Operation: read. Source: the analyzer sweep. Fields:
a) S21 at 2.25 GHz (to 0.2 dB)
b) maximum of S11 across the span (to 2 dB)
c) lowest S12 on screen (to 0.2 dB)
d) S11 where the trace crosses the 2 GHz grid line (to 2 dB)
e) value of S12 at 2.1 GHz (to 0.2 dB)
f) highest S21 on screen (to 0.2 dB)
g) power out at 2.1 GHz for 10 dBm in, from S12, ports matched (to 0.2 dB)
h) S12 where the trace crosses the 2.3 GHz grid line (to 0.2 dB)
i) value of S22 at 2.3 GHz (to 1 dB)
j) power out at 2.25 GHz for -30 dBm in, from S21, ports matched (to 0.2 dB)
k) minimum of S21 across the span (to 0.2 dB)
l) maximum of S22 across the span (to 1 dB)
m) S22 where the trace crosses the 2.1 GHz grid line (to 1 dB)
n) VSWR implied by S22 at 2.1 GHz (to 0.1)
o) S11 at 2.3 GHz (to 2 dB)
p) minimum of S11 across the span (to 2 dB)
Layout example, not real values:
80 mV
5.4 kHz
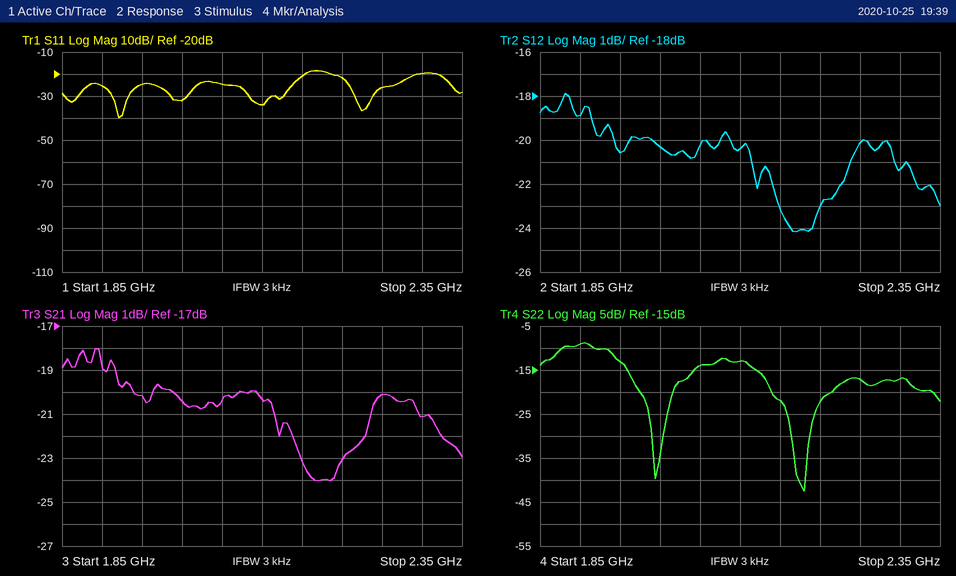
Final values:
-20.2 dB
-18 dB
-24.2 dB
-32 dB
-20.4 dB
-18.0 dB
-10.4 dBm
-21.4 dB
-17 dB
-50.2 dBm
-24.0 dB
-9 dB
-13 dB
1.6
-20 dB
-40 dB
